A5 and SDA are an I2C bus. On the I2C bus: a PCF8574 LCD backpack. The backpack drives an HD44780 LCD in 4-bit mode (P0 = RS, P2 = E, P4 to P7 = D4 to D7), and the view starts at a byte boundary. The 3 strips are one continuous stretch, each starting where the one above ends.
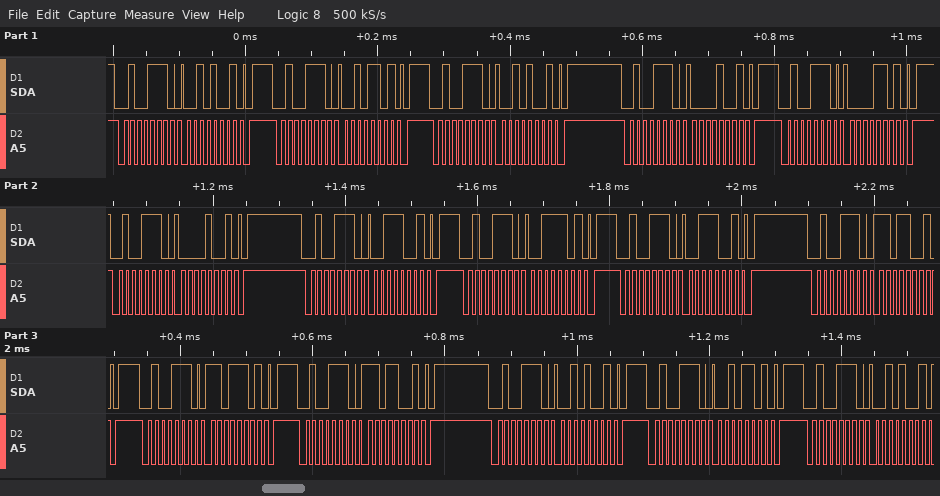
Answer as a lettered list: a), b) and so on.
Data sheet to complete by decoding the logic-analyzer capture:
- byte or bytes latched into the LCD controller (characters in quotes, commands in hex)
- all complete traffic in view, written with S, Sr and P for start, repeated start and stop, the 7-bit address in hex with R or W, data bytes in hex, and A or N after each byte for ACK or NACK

a) ' ' '='
b) S 27W A 29 A P S 27W A 2D A P S 27W A 29 A P S 27W A 09 A P S 27W A 0D A P S 27W A 09 A P S 27W A 39 A P S 27W A 3D A P S 27W A 39 A P S 27W A D9 A P S 27W A DD A P S 27W A D9 A P S 27W A 29 A P S 27W A 2D A P S 27W A 29 A
